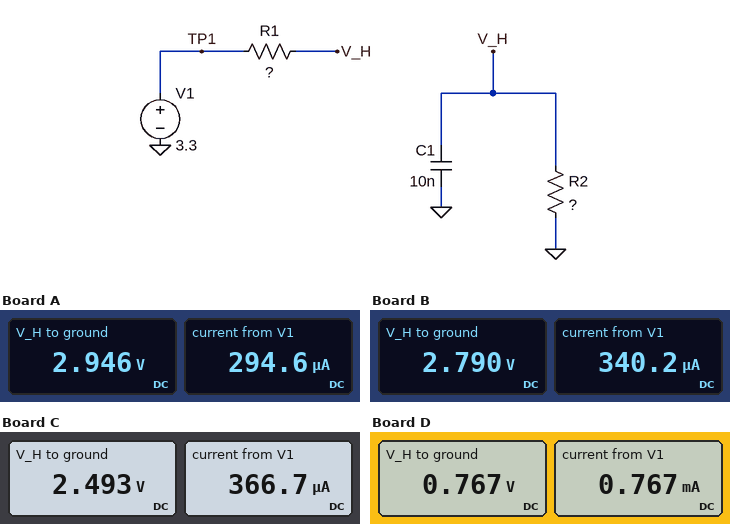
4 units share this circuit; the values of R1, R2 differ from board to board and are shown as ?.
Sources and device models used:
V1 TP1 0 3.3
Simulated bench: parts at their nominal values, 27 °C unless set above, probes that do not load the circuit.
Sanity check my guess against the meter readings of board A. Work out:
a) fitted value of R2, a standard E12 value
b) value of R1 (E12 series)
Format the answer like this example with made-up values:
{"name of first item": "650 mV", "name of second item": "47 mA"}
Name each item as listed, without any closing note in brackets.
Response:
{"fitted value of R2, a standard E12 value": "10 kΩ", "value of R1": "1.2 kΩ"}
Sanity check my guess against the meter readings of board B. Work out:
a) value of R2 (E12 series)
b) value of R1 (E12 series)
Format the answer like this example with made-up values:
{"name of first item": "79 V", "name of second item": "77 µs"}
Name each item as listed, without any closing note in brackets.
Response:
{"value of R2": "8.2 kΩ", "value of R1": "1.5 kΩ"}
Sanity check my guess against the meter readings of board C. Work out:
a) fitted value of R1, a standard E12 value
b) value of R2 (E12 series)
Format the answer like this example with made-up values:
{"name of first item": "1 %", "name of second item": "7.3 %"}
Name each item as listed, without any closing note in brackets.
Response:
{"fitted value of R1, a standard E12 value": "2.2 kΩ", "value of R2": "6.8 kΩ"}
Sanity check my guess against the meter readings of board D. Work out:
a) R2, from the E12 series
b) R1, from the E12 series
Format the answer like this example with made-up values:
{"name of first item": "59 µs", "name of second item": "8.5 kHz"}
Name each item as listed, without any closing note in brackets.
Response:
{"R2, from the E12 series": "1 kΩ", "R1, from the E12 series": "3.3 kΩ"}
